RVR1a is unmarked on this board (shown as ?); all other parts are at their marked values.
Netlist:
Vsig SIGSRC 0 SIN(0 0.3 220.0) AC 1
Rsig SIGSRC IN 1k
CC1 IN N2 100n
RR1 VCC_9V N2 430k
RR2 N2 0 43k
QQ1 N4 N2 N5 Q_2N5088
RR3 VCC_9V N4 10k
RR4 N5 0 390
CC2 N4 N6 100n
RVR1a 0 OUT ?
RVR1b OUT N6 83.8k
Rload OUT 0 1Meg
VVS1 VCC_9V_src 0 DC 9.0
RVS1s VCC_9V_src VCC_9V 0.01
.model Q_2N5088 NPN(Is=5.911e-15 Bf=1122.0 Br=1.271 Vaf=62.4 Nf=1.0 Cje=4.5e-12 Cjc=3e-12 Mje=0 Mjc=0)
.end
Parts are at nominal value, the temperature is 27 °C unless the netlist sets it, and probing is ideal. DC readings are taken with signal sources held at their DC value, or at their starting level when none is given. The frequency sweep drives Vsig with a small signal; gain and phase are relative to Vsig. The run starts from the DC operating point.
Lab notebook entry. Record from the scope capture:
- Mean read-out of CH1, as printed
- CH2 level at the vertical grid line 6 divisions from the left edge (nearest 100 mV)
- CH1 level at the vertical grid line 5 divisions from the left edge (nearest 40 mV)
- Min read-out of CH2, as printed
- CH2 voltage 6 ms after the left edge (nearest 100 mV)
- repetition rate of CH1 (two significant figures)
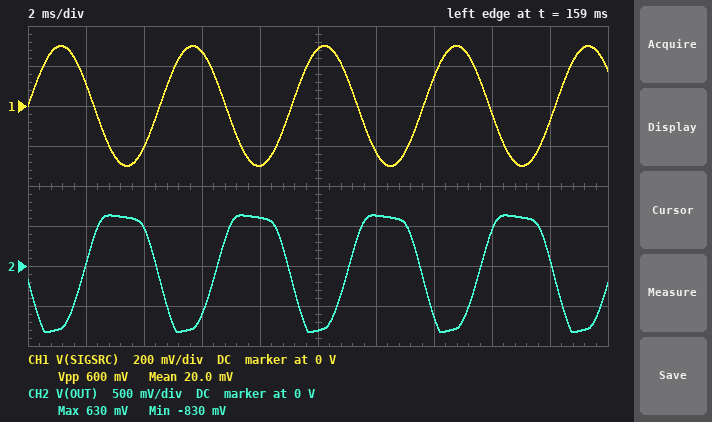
20.0 mV
600 mV
280 mV
-830 mV
-600 mV
220 Hz
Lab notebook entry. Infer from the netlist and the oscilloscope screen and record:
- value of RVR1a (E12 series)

18 kΩ
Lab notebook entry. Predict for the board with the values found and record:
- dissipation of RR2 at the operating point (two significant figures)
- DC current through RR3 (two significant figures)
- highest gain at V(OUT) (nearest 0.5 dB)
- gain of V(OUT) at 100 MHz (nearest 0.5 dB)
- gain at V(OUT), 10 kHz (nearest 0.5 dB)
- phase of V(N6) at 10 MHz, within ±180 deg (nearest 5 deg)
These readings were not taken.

15 µW
410 µA
10.5 dB
-21.5 dB
10.5 dB
95 deg
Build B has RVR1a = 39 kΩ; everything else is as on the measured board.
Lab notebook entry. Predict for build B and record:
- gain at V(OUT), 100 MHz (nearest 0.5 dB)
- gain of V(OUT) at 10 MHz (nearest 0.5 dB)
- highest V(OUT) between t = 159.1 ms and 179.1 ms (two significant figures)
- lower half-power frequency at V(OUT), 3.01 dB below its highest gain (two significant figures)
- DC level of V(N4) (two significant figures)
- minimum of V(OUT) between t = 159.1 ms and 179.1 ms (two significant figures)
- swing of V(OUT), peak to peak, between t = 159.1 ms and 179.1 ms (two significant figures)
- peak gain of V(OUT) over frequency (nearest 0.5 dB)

-16.5 dB
0.5 dB
1.1 V
46 Hz
4.9 V
-1.5 V
2.6 V
15.5 dB
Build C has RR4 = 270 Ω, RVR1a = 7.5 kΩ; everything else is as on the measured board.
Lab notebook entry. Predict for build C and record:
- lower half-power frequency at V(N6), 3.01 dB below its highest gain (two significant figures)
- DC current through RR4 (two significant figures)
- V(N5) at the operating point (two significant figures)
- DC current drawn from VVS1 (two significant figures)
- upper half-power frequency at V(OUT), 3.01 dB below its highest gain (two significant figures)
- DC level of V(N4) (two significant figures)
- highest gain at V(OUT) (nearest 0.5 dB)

49 Hz
550 µA
150 mV
570 µA
1.4 MHz
3.5 V
7.0 dB
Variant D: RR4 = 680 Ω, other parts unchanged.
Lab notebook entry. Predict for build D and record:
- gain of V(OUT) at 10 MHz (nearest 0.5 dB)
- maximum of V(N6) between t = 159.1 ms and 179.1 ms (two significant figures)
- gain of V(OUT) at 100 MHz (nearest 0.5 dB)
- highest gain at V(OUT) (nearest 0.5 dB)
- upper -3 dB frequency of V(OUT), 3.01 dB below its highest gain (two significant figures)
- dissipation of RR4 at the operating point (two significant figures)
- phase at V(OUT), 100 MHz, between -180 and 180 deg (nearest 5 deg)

-6.5 dB
2.6 V
-20.5 dB
6.0 dB
2.5 MHz
47 µW
30 deg
